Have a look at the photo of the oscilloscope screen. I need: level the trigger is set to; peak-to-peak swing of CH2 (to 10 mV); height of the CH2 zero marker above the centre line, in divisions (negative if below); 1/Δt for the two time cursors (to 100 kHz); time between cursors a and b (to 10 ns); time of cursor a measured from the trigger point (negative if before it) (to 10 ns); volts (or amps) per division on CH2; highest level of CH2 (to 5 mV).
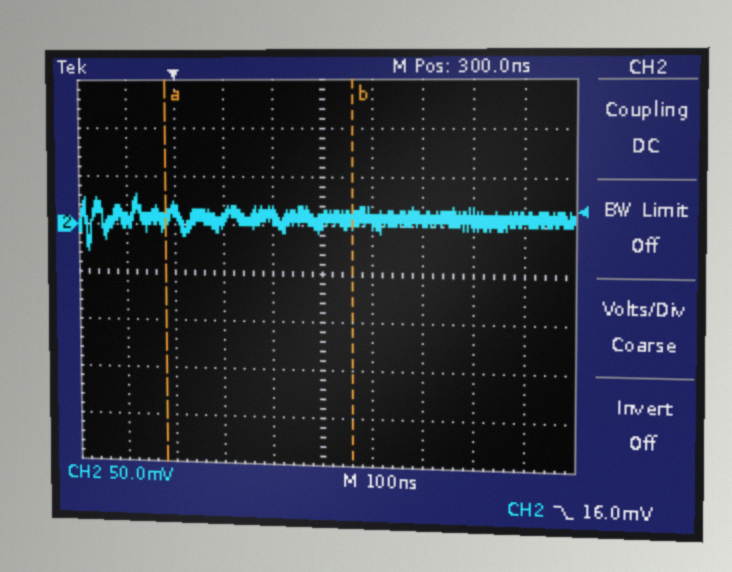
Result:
16.0 mV
60 mV
+1.0 div
2.6 MHz
380 ns
-20 ns
50 mV
30 mV
